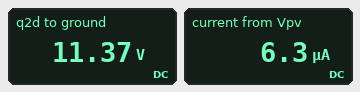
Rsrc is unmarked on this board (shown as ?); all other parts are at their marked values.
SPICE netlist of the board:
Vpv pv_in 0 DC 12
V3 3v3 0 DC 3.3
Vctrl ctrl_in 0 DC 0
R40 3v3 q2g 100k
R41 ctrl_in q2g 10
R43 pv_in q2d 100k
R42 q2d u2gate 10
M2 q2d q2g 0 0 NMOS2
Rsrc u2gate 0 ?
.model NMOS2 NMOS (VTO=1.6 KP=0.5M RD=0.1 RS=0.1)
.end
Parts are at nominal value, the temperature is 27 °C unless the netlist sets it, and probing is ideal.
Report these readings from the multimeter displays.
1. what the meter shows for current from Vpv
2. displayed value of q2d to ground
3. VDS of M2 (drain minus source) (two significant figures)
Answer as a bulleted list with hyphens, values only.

- 6.3 µA
- 11.37 V
- 11 V
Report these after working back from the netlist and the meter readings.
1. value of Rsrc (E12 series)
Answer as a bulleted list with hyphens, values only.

- 1.8 MΩ
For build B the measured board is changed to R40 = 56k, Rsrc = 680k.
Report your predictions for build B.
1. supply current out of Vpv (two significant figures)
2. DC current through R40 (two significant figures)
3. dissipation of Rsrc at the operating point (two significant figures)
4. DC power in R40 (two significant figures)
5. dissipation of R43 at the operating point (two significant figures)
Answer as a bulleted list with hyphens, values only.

- 15 µA
- 59 µA
- 160 µW
- 190 µW
- 24 µW
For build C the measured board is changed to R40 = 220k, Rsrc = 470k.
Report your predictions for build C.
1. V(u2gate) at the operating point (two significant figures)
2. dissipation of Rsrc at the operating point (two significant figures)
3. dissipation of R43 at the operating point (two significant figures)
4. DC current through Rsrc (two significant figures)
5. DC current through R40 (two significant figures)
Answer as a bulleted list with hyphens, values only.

- 9.9 V
- 210 µW
- 44 µW
- 21 µA
- 15 µA
